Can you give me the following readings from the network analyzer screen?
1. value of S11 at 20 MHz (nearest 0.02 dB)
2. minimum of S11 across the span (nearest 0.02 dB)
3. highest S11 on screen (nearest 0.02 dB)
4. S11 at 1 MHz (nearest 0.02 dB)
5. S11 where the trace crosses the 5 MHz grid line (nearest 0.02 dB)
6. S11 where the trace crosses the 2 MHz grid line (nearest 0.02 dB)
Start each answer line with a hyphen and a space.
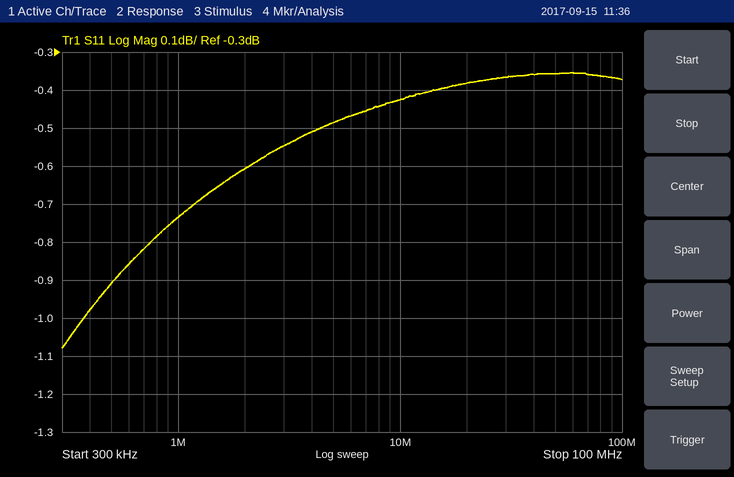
- -0.38 dB
- -1.08 dB
- -0.36 dB
- -0.74 dB
- -0.48 dB
- -0.60 dB
